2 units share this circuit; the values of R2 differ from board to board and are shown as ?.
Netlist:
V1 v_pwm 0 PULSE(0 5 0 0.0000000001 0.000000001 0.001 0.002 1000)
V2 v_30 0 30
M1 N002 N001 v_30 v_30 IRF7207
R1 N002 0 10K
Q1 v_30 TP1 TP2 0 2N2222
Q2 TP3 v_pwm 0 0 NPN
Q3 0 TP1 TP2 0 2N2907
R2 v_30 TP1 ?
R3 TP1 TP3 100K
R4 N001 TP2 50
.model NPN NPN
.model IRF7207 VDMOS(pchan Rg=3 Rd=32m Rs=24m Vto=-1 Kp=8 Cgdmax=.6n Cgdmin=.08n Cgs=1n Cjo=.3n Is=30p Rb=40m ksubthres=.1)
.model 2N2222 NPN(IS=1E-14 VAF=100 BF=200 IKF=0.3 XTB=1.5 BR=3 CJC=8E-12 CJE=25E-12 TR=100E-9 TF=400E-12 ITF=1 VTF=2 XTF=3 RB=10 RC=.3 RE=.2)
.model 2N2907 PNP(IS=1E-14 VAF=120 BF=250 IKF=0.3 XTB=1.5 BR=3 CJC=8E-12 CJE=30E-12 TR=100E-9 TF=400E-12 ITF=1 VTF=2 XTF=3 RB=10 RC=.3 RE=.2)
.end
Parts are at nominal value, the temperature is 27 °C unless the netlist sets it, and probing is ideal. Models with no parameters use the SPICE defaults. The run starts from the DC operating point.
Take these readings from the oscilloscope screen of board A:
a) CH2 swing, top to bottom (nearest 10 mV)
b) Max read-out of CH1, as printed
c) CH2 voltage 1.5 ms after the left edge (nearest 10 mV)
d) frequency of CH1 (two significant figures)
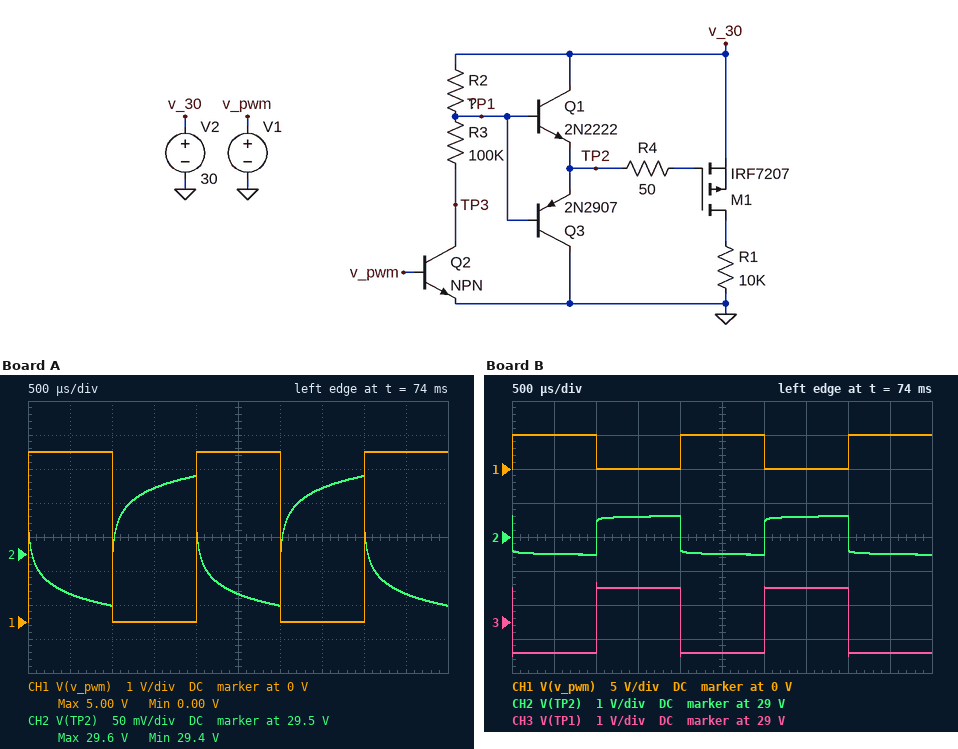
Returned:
190 mV
5.00 V
29.60 V
500 Hz
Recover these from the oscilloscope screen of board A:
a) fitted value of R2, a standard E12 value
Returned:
3.3 kΩ
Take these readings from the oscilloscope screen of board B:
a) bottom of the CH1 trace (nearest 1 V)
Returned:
0 V
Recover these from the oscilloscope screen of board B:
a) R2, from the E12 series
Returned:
6.8 kΩ
